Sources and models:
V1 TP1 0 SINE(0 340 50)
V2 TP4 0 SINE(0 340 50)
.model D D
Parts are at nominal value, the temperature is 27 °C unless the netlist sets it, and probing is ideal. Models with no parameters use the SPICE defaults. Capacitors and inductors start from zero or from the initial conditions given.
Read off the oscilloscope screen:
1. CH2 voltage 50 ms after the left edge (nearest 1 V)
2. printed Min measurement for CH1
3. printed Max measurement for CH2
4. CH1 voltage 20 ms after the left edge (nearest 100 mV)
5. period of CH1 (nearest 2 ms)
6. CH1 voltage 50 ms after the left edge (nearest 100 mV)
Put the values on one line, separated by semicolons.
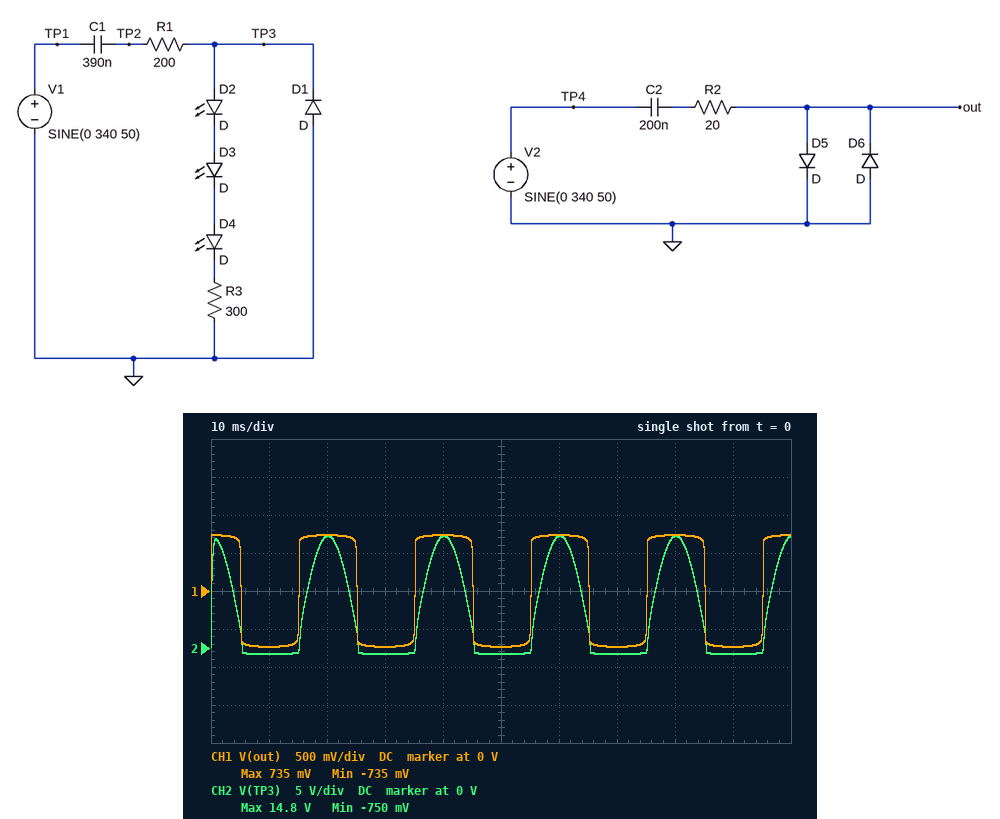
-1 V; -735 mV; 14.8 V; 700 mV; 20 ms; -700 mV
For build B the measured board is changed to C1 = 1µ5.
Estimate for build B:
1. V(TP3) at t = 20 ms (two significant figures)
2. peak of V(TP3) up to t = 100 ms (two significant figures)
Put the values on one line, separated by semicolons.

48 V; 49 V
